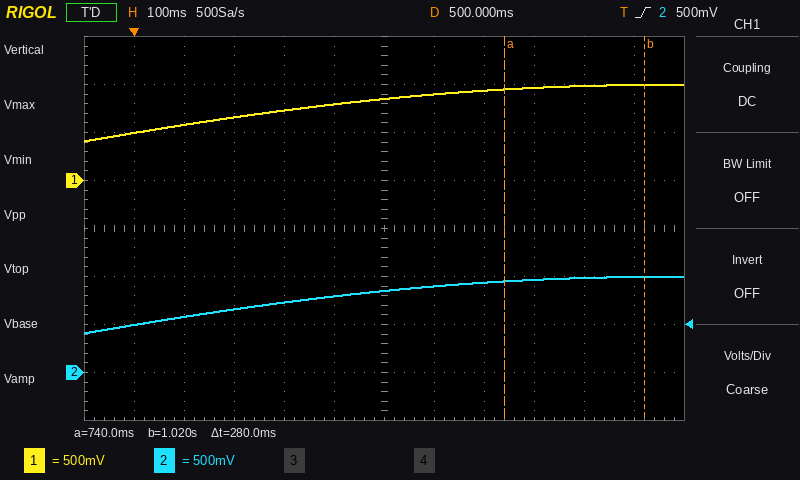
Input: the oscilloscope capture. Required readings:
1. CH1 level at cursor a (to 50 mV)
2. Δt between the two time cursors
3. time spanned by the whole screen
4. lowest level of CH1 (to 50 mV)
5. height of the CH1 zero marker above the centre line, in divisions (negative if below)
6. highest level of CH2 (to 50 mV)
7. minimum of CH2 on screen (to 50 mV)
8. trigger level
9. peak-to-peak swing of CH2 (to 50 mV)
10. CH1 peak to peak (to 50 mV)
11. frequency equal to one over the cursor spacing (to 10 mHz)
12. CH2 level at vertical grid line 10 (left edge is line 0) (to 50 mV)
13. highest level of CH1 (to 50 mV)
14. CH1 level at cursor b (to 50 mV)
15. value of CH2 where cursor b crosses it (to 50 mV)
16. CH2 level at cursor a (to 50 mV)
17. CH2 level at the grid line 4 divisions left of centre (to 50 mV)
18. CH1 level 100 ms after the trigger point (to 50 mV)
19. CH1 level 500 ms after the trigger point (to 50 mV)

950 mV
280 ms
1.2 s
400 mV
+1.0 div
1.00 V
400 mV
500 mV
600 mV
600 mV
3.57 Hz
1.00 V
1.00 V
1.00 V
1.00 V
950 mV
600 mV
600 mV
850 mV
